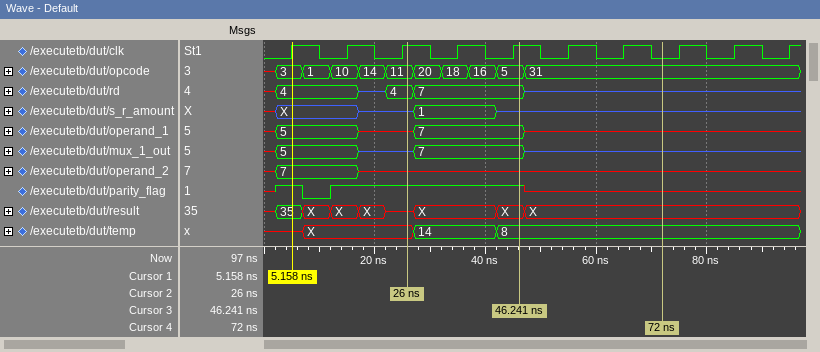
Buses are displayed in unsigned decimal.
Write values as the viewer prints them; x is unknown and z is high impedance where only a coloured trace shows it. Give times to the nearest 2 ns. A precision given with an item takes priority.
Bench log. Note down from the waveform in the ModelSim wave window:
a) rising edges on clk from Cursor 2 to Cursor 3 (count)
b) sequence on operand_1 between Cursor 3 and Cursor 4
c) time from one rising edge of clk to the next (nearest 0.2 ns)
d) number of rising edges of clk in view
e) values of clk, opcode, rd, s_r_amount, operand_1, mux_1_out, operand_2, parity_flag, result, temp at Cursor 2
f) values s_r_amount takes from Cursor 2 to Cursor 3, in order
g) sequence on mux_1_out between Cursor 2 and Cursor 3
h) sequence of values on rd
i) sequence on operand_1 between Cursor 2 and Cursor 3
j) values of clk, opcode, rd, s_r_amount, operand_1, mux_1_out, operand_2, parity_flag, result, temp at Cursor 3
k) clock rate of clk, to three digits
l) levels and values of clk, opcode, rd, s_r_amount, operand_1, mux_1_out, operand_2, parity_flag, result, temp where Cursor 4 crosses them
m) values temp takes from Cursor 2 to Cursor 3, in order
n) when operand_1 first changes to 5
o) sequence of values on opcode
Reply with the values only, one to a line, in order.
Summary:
2
7, x
10 ns
10
clk=1, opcode=11, rd=4, s_r_amount=z, operand_1=x, mux_1_out=z, operand_2=x, parity_flag=1, result=x, temp=X
z, 1, z
z, 7
x, 4, z, 4, 7, z
x, 7
clk=1, opcode=5, rd=7, s_r_amount=z, operand_1=7, mux_1_out=7, operand_2=x, parity_flag=1, result=X, temp=8
100 MHz
clk=0, opcode=31, rd=z, s_r_amount=z, operand_1=x, mux_1_out=z, operand_2=x, parity_flag=x, result=X, temp=8
X, 14, 8
2 ns
x, 3, 1, 10, 14, 11, 20, 18, 16, 5, 31
